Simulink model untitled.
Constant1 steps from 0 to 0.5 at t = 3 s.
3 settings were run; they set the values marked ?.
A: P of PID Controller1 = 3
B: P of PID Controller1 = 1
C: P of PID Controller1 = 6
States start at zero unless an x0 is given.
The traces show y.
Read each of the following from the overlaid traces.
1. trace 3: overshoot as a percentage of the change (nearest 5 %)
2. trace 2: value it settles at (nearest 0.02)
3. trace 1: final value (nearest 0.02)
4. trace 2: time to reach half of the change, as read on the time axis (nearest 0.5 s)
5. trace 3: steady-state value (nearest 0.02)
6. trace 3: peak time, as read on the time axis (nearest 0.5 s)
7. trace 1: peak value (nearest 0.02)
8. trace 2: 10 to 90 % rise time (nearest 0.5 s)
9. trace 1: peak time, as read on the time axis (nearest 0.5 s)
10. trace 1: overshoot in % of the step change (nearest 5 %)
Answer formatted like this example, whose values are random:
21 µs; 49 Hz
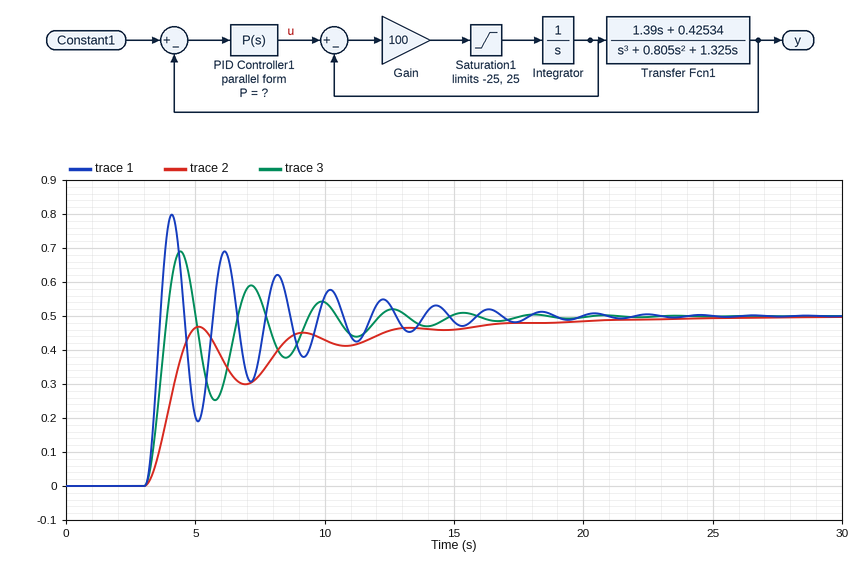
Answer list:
40 %; 0.50; 0.50; 4.0 s; 0.50; 4.5 s; 0.80; 1.5 s; 4.0 s; 60 %
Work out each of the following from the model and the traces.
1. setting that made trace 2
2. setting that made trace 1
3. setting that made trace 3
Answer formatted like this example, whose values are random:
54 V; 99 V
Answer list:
B; C; A
